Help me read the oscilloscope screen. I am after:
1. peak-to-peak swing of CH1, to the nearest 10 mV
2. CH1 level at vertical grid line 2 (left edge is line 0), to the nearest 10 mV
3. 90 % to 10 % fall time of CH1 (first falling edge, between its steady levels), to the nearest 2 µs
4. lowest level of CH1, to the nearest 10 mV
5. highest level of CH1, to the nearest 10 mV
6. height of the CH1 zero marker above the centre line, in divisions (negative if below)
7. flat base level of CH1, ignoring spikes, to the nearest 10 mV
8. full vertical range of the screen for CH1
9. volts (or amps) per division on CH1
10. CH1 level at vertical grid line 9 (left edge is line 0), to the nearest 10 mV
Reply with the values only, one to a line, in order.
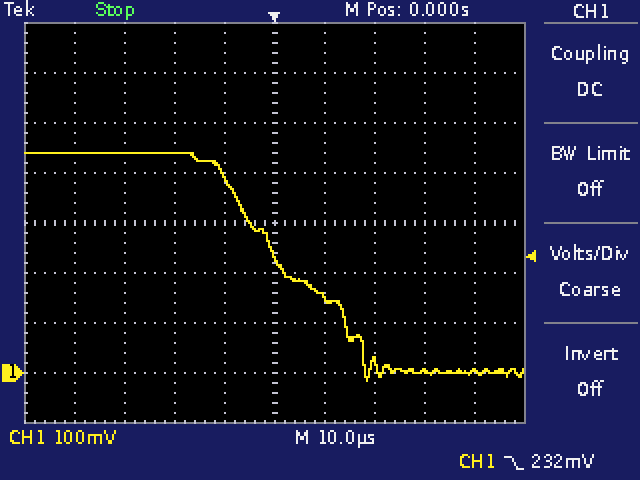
460 mV
440 mV
28 µs
-20 mV
440 mV
-3.0 div
0 mV
800 mV
100 mV
0 mV
